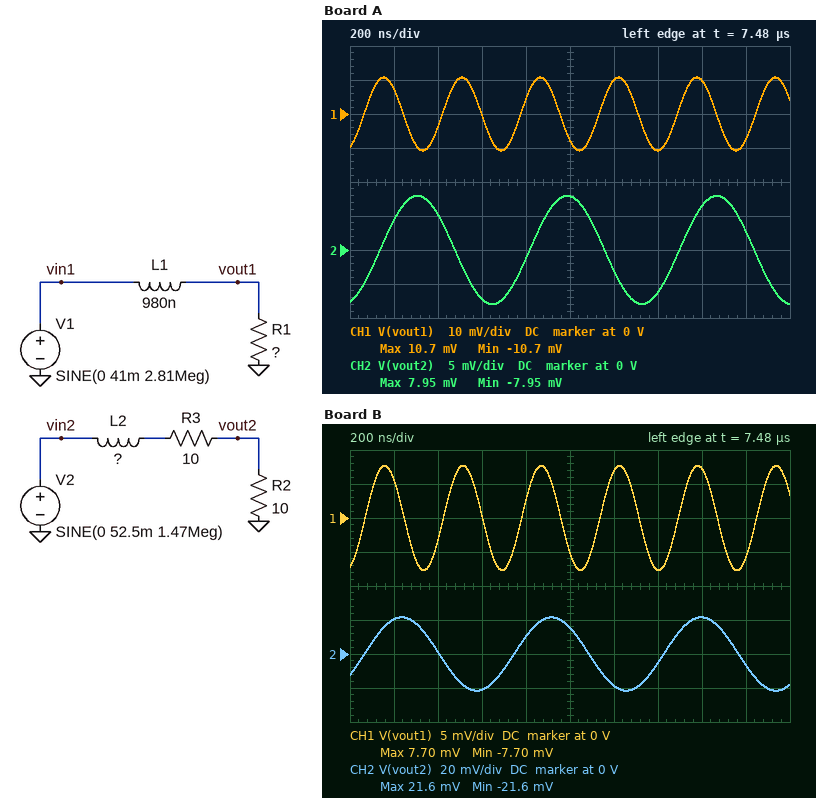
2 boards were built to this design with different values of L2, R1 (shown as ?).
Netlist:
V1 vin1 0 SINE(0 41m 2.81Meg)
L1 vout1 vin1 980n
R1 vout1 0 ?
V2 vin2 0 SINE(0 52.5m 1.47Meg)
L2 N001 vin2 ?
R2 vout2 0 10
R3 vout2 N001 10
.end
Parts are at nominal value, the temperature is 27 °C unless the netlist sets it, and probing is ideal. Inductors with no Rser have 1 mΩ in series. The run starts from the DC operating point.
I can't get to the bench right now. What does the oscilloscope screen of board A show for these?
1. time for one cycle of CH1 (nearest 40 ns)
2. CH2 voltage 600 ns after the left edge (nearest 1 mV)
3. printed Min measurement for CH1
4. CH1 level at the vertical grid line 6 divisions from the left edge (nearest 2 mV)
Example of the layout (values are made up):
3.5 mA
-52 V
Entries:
360 ns
-7 mV
-10.7 mV
10 mV
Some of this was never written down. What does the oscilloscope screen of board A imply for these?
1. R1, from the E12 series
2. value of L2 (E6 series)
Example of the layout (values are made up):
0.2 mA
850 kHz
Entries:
4.7 Ω
6.8 µH
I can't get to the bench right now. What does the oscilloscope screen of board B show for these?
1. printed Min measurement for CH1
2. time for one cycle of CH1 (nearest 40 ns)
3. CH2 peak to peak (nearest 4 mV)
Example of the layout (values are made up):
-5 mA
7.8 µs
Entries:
-7.70 mV
360 ns
44 mV
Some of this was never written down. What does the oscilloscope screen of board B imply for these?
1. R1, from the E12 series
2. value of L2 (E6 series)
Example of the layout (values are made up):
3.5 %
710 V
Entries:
3.3 Ω
1.5 µH
